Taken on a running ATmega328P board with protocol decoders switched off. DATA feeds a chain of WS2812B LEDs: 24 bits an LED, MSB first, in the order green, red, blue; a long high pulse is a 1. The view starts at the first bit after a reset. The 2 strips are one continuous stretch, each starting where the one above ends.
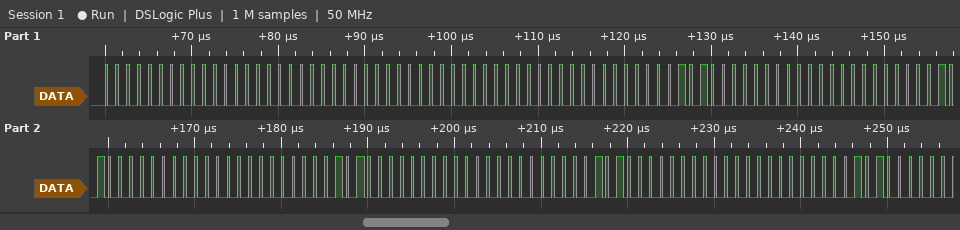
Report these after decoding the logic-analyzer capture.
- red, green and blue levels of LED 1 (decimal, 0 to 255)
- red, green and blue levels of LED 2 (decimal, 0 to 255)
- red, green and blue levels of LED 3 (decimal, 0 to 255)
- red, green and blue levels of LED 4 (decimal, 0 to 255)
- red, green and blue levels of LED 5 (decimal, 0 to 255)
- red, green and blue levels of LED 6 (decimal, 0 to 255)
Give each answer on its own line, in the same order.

0, 0, 0
0, 0, 0
0, 5, 0
0, 5, 0
0, 5, 0
0, 5, 0
